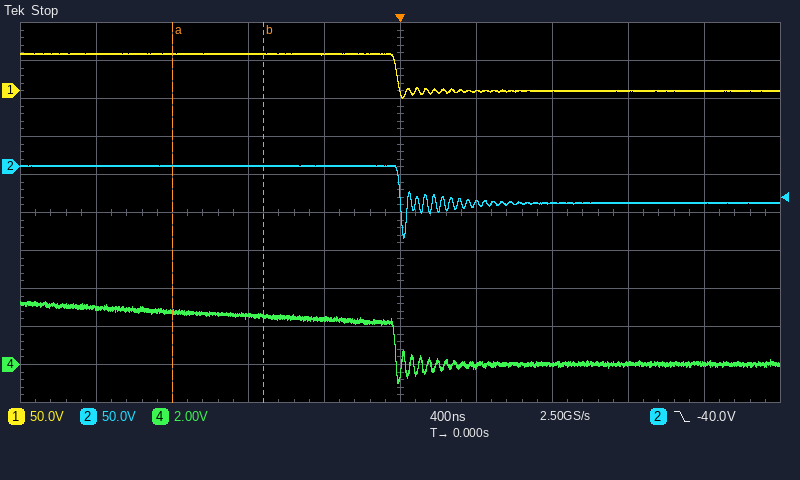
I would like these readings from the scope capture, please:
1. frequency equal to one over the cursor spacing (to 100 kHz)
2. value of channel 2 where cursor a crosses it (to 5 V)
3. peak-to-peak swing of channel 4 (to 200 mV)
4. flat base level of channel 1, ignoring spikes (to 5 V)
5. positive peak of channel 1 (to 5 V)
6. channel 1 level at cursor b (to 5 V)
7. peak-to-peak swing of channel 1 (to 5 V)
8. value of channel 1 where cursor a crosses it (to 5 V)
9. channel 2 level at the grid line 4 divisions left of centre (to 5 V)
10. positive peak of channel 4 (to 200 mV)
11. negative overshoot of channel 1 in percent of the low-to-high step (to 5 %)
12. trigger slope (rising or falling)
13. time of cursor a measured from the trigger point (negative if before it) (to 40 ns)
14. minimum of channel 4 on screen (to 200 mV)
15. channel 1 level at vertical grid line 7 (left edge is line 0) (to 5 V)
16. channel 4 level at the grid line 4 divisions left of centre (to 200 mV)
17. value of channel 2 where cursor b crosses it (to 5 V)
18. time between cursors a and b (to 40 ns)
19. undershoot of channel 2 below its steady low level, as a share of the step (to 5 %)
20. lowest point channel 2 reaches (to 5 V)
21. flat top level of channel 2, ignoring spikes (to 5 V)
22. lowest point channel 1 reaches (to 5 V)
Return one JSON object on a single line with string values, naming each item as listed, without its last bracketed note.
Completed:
{"frequency equal to one over the cursor spacing": "2.1 MHz", "value of channel 2 where cursor a crosses it": "0 V", "peak-to-peak swing of channel 4": "4.4 V", "flat base level of channel 1, ignoring spikes": "0 V", "positive peak of channel 1": "50 V", "channel 1 level at cursor b": "50 V", "peak-to-peak swing of channel 1": "60 V", "value of channel 1 where cursor a crosses it": "50 V", "channel 2 level at the grid line 4 divisions left of centre": "0 V", "positive peak of channel 4": "3.4 V", "negative overshoot of channel 1 in percent of the low-to-high step": "20 %", "trigger slope": "falling", "time of cursor a measured from the trigger point (negative if before it)": "-1.20 µs", "minimum of channel 4 on screen": "-1.0 V", "channel 1 level at vertical grid line 7 (left edge is line 0)": "0 V", "channel 4 level at the grid line 4 divisions left of centre": "3.0 V", "value of channel 2 where cursor b crosses it": "0 V", "time between cursors a and b": "480 ns", "undershoot of channel 2 below its steady low level, as a share of the step": "95 %", "lowest point channel 2 reaches": "-95 V", "flat top level of channel 2, ignoring spikes": "0 V", "lowest point channel 1 reaches": "-10 V"}
